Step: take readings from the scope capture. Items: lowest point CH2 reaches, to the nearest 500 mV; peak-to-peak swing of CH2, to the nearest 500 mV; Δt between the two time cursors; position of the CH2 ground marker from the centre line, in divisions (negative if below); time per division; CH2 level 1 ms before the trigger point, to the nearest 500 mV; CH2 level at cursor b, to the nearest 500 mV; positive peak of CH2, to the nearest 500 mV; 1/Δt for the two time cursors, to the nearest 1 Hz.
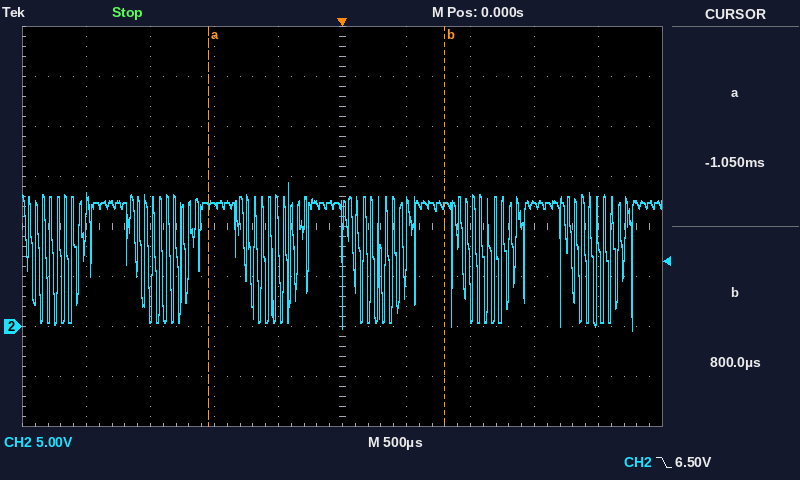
-500 mV
15.0 V
1.85 ms
-2.0 div
500 µs
12.0 V
12.0 V
14.5 V
541 Hz
